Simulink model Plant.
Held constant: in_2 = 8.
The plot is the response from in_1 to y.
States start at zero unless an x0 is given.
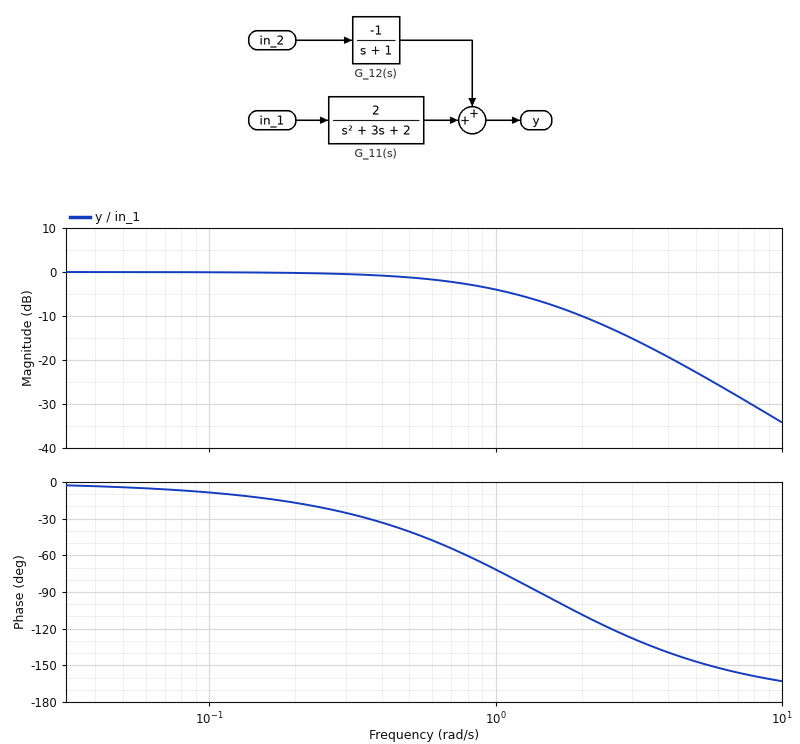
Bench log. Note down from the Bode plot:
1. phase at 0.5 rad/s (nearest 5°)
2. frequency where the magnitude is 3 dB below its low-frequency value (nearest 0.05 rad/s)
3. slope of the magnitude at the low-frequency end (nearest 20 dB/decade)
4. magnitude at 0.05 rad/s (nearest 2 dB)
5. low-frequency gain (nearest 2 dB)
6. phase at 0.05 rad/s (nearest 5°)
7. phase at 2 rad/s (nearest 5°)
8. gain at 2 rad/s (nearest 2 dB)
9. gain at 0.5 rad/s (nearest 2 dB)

-40°
0.85 rad/s
0 dB/decade
0 dB
0 dB
-5°
-110°
-10 dB
-2 dB
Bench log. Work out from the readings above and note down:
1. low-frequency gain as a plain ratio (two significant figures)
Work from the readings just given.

1.0
